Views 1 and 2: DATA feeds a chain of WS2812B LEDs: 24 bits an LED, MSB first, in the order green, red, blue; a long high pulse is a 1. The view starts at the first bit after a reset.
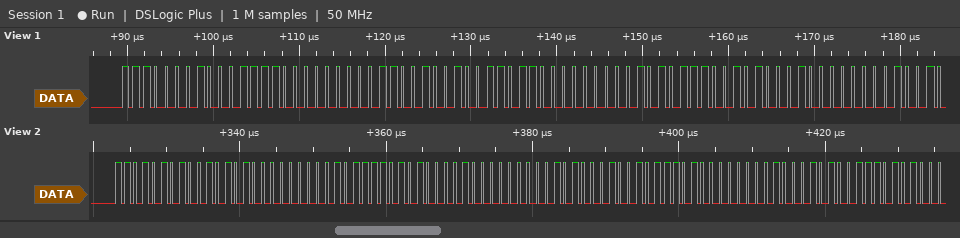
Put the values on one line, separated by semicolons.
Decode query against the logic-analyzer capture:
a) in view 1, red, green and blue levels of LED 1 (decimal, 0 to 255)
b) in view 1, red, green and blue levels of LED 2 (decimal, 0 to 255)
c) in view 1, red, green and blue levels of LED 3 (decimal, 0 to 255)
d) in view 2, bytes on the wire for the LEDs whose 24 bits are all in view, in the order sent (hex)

30, 225, 0; 54, 201, 0; 81, 174, 0; D5 2A 00 BD 42 00 A2 5D 00
